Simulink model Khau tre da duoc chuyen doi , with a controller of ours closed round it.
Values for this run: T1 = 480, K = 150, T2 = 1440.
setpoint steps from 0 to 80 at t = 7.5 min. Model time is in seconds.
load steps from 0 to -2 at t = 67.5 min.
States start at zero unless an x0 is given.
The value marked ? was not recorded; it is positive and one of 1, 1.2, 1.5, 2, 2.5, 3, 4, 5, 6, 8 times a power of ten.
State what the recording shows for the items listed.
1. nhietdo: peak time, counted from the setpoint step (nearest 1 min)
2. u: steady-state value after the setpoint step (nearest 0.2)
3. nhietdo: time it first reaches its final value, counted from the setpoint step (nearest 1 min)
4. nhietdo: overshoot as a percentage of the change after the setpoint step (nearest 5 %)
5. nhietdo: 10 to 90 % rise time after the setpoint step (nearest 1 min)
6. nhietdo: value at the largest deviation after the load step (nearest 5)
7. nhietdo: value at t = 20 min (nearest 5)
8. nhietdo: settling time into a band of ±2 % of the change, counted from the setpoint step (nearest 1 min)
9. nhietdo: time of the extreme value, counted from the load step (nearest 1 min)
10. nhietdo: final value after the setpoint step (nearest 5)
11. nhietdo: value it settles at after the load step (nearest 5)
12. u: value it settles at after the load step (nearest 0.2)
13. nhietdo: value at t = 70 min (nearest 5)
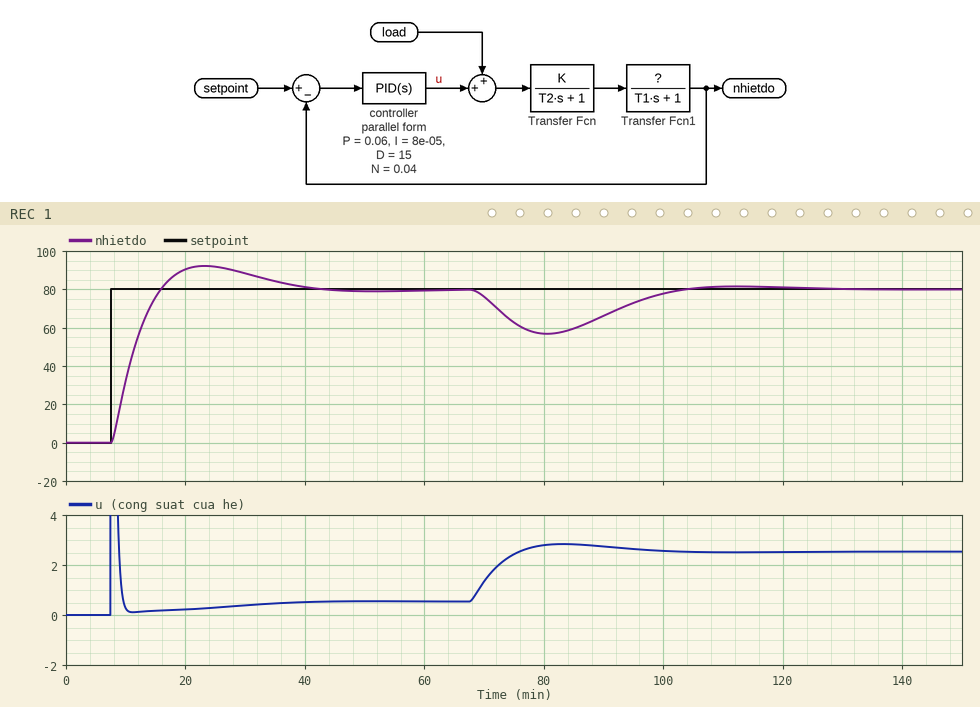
16 min
0.6
8 min
15 %
6 min
55
90
32 min
13 min
80
80
2.6
75
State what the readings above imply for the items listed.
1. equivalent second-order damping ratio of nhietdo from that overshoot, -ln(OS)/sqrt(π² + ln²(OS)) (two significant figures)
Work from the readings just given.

0.52
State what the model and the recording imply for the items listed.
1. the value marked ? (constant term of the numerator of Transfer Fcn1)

1
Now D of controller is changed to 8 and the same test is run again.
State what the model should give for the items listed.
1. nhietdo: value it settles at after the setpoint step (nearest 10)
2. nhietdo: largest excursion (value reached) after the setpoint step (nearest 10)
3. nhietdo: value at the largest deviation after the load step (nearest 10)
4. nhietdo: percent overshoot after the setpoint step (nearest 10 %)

80
100
50
30 %
